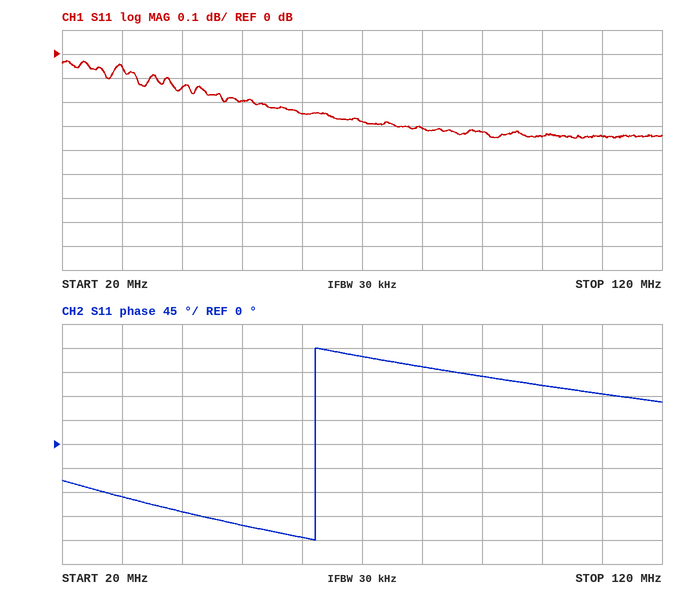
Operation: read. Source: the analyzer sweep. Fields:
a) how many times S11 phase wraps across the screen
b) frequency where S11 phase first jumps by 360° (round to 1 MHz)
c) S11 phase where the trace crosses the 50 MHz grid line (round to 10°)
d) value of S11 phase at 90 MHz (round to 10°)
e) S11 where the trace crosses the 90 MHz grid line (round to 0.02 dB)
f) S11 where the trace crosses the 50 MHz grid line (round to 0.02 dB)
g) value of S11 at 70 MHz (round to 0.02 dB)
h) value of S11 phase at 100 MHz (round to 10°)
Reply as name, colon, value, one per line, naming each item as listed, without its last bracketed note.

how many times S11 phase wraps across the screen: 1
frequency where S11 phase first jumps by 360°: 62 MHz
S11 phase where the trace crosses the 50 MHz grid line: -150°
value of S11 phase at 90 MHz: 130°
S11 where the trace crosses the 90 MHz grid line: -0.32 dB
S11 where the trace crosses the 50 MHz grid line: -0.20 dB
value of S11 at 70 MHz: -0.28 dB
value of S11 phase at 100 MHz: 110°
